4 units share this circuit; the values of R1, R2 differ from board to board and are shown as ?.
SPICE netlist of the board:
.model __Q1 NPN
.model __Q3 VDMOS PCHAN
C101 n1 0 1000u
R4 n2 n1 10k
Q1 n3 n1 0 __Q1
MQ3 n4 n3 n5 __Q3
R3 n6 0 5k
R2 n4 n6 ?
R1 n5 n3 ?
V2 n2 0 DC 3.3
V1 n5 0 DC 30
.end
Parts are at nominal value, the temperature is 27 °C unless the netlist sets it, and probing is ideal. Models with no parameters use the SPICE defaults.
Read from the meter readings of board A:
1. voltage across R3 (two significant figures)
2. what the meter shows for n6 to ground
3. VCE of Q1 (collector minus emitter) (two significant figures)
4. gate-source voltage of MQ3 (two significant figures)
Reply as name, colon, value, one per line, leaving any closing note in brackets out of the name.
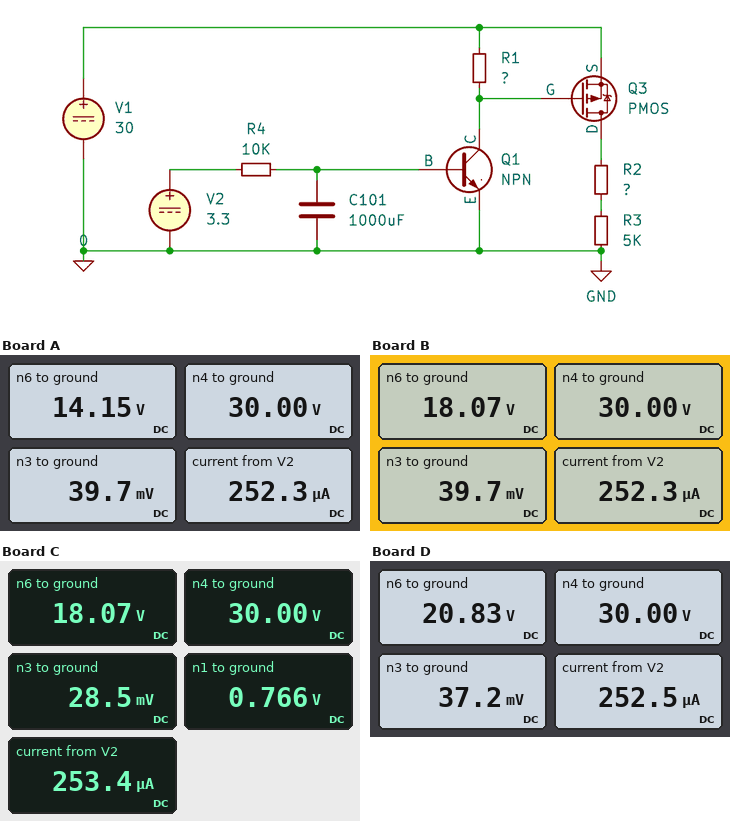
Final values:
voltage across R3: 14 V
what the meter shows for n6 to ground: 14.15 V
VCE of Q1 (collector minus emitter): 40 mV
gate-source voltage of MQ3: -30 V
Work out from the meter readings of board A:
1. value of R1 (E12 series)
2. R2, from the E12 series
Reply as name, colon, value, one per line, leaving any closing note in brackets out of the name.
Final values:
value of R1: 47 kΩ
R2, from the E12 series: 5.6 kΩ
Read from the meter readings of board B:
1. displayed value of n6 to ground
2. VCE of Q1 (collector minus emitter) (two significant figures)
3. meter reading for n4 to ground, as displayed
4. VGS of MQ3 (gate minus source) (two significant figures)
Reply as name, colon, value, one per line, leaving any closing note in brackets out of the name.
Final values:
displayed value of n6 to ground: 18.07 V
VCE of Q1 (collector minus emitter): 40 mV
meter reading for n4 to ground, as displayed: 30.00 V
VGS of MQ3 (gate minus source): -30 V
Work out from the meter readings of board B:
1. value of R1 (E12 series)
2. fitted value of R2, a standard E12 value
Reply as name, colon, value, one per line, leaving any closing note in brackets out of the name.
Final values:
value of R1: 47 kΩ
fitted value of R2, a standard E12 value: 3.3 kΩ
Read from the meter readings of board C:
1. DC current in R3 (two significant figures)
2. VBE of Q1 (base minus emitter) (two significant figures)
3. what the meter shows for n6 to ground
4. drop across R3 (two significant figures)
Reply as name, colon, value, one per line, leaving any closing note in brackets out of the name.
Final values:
DC current in R3: 3.6 mA
VBE of Q1 (base minus emitter): 770 mV
what the meter shows for n6 to ground: 18.07 V
drop across R3: 18 V
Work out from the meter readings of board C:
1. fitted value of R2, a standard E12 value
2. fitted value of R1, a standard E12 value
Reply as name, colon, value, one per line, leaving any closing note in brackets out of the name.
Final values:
fitted value of R2, a standard E12 value: 3.3 kΩ
fitted value of R1, a standard E12 value: 120 kΩ
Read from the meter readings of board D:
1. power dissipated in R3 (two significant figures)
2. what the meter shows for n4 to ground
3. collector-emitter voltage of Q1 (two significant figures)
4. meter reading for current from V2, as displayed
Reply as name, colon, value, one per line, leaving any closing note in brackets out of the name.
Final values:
power dissipated in R3: 87 mW
what the meter shows for n4 to ground: 30.00 V
collector-emitter voltage of Q1: 37 mV
meter reading for current from V2, as displayed: 252.5 µA
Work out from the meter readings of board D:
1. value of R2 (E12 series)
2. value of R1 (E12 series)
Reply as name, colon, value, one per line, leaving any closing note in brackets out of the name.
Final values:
value of R2: 2.2 kΩ
value of R1: 56 kΩ
